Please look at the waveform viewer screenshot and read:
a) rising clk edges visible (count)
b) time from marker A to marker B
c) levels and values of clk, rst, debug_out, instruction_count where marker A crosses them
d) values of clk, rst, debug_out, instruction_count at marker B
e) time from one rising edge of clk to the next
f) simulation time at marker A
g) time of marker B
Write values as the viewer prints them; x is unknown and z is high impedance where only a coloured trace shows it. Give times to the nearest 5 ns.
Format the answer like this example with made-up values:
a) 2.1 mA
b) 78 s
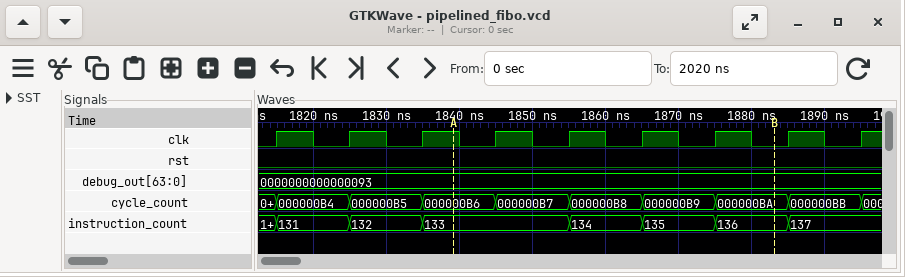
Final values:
a) 9
b) 45 ns
c) clk=1, rst=0, debug_out=0000000000000093, instruction_count=133
d) clk=0, rst=0, debug_out=0000000000000093, instruction_count=136
e) 10 ns
f) 1840 ns
g) 1885 ns
